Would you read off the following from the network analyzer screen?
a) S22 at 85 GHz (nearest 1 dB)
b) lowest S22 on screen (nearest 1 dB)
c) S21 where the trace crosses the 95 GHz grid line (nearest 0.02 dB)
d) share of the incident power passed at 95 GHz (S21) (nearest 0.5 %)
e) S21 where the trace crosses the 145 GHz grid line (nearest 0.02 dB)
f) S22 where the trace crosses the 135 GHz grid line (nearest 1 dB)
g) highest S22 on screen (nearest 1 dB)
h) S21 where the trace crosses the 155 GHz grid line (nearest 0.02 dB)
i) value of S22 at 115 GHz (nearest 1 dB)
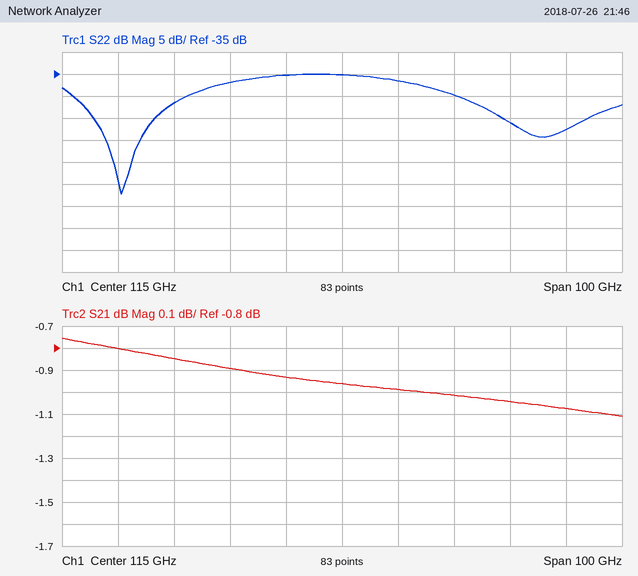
-42 dB
-62 dB
-0.90 dB
81.5 %
-1.04 dB
-40 dB
-35 dB
-1.08 dB
-35 dB
